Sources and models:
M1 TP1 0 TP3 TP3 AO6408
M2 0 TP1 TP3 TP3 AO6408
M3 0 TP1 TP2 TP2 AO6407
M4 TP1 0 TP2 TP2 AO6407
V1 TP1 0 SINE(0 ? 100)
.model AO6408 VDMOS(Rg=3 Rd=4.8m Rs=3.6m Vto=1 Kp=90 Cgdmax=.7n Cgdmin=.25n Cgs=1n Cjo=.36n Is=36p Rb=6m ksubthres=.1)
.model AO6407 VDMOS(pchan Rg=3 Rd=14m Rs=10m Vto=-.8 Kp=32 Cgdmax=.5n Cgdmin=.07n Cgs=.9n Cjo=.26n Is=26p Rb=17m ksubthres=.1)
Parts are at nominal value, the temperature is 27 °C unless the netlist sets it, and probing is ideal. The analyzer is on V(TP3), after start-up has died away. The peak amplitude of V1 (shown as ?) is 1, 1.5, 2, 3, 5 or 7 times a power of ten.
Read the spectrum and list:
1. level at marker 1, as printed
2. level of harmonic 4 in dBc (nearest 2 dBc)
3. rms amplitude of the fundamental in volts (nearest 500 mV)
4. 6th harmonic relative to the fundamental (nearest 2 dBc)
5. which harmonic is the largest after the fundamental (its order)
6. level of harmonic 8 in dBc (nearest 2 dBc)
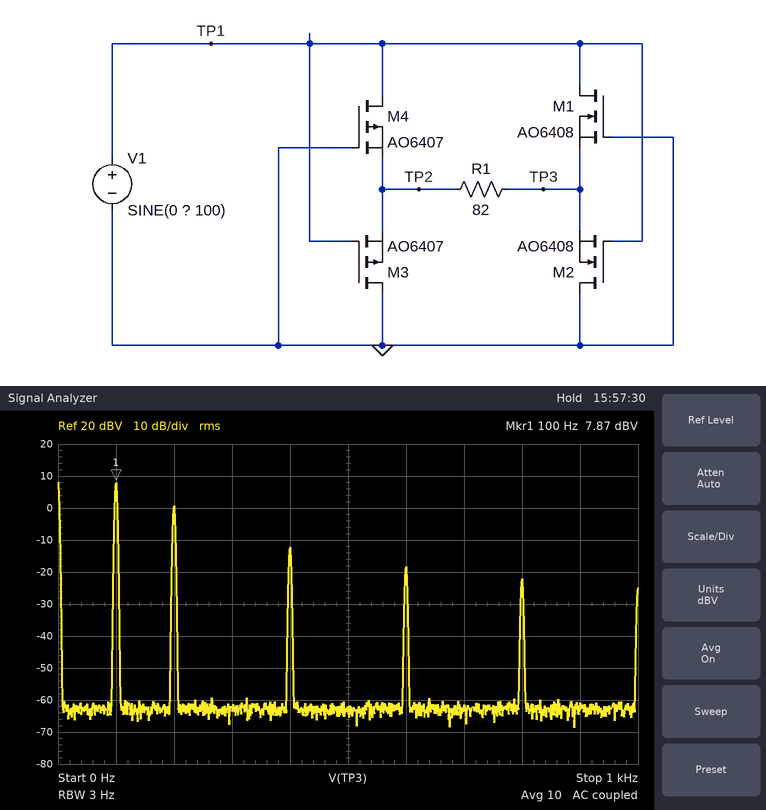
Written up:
7.87 dBV
-20 dBc
2.5 V
-26 dBc
2
-30 dBc
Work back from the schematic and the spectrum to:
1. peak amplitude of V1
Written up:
7 V
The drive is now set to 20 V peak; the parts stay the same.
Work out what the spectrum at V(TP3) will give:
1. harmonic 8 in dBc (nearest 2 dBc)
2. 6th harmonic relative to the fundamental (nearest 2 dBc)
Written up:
-34 dBc
-28 dBc
